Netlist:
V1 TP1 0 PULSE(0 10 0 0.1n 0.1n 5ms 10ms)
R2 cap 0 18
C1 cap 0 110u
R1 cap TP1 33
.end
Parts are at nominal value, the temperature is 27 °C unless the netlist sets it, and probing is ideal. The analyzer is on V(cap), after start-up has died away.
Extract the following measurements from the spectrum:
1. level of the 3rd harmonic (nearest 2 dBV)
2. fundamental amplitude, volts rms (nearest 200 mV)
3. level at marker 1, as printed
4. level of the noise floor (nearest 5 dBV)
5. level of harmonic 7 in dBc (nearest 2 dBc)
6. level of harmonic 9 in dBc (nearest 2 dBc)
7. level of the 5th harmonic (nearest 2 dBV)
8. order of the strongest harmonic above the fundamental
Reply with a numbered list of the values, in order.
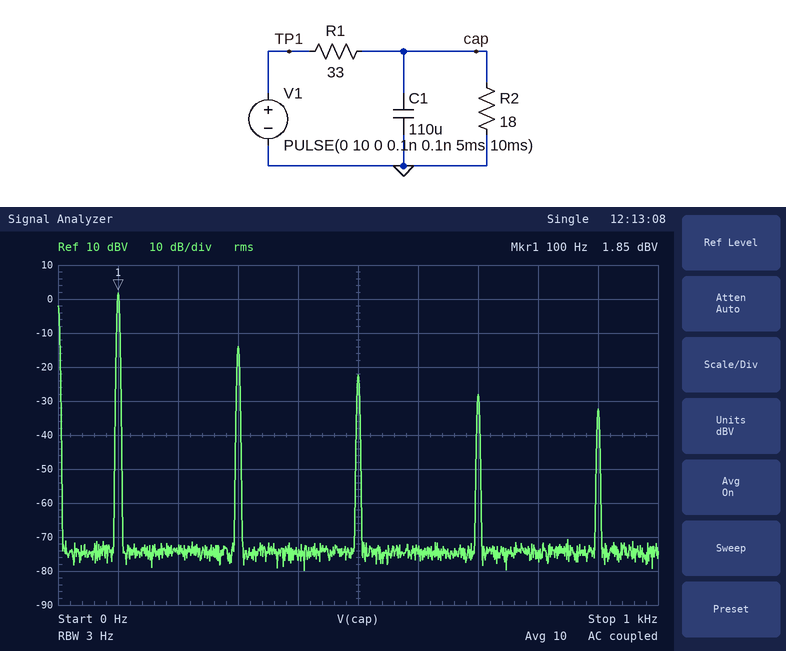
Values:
1. -14 dBV
2. 1.2 V
3. 1.85 dBV
4. -75 dBV
5. -30 dBc
6. -34 dBc
7. -22 dBV
8. 3
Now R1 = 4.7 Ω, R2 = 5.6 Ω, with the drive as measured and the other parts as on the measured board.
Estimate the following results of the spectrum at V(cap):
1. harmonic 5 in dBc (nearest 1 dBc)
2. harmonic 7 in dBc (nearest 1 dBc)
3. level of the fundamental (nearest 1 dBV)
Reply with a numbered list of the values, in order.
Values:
1. -16 dBc
2. -21 dBc
3. 8 dBV
